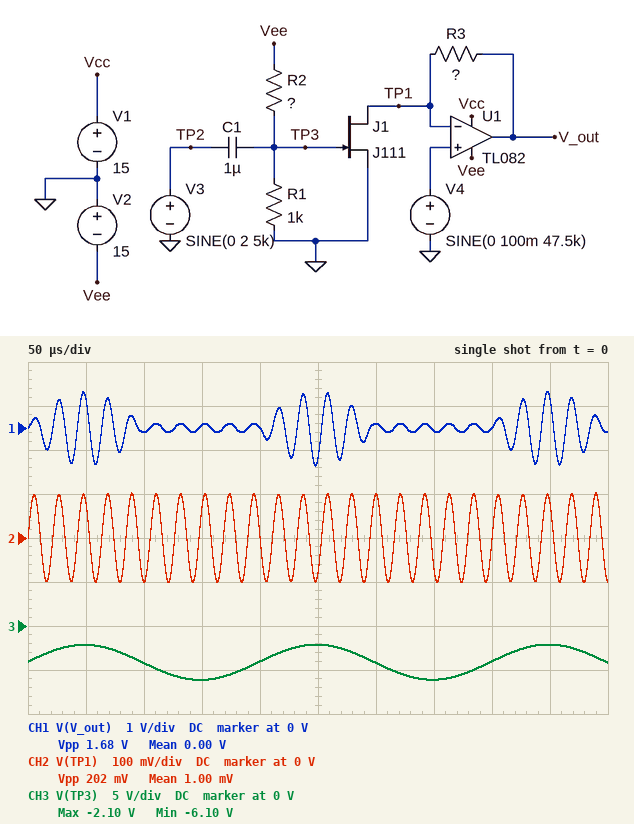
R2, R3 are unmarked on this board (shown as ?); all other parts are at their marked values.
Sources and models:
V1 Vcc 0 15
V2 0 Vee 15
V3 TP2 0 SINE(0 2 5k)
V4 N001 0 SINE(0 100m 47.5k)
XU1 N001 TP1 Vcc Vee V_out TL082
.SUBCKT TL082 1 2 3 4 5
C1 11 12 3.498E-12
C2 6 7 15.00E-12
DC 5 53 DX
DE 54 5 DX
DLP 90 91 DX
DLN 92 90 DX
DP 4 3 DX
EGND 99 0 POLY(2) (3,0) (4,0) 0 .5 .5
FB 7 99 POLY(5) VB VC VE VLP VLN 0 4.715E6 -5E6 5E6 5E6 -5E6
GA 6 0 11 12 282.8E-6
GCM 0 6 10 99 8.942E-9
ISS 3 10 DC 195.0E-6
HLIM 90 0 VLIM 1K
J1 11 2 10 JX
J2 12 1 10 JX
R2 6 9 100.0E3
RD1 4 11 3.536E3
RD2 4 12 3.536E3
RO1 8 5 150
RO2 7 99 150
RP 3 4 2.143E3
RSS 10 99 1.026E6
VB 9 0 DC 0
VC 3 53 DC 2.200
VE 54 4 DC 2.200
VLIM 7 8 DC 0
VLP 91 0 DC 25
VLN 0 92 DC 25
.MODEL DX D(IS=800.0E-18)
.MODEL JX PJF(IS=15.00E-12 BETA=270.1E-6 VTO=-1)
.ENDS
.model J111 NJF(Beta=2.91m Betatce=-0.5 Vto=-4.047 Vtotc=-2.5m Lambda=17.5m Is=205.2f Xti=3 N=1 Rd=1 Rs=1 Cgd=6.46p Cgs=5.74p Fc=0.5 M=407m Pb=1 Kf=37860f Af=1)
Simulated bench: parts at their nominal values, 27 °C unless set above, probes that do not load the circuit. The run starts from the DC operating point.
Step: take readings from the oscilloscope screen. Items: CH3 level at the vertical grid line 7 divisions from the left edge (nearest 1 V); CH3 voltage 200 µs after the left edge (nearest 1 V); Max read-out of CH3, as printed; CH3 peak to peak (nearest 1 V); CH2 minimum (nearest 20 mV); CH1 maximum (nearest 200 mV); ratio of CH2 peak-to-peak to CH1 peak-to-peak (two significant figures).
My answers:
-6 V
-4 V
-2.10 V
4 V
-100 mV
800 mV
0.12
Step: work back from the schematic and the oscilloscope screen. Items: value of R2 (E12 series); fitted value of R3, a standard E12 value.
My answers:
2.7 kΩ
680 Ω
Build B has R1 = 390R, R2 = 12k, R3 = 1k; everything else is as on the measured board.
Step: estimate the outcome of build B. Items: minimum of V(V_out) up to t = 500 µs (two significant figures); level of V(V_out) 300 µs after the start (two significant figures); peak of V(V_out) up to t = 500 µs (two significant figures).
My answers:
-13 V
1.5 V
2.4 V
